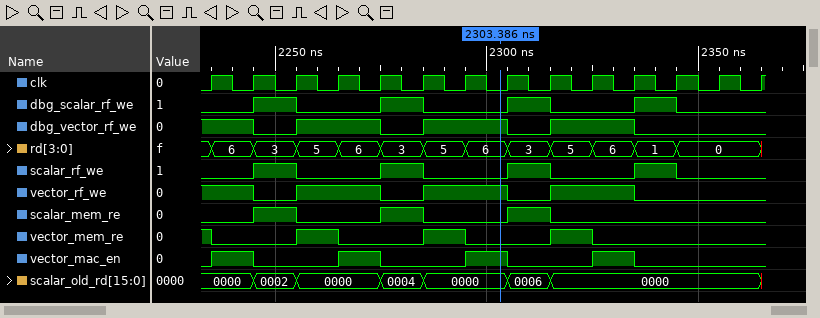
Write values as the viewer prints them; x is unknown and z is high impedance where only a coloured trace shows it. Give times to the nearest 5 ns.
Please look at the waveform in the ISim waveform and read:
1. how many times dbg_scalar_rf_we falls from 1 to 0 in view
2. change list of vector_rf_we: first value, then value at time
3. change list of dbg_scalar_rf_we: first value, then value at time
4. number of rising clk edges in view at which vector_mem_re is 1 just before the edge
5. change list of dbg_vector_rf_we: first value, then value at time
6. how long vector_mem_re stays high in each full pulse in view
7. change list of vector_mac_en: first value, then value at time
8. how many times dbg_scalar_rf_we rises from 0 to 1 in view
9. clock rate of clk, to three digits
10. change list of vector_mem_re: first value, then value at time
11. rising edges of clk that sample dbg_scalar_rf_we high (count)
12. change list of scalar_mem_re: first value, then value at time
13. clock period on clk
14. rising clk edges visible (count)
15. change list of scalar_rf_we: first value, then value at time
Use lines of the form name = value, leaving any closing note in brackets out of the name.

how many times dbg_scalar_rf_we falls from 1 to 0 in view = 4
change list of vector_rf_we: first value, then value at time = 1, 0 at 2245 ns, 1 at 2255 ns, 0 at 2275 ns, 1 at 2285 ns, 0 at 2305 ns, 1 at 2315 ns, 0 at 2335 ns
change list of dbg_scalar_rf_we: first value, then value at time = 0, 1 at 2245 ns, 0 at 2255 ns, 1 at 2275 ns, 0 at 2285 ns, 1 at 2305 ns, 0 at 2315 ns, 1 at 2335 ns, 0 at 2345 ns
number of rising clk edges in view at which vector_mem_re is 1 just before the edge = 4
change list of dbg_vector_rf_we: first value, then value at time = 1, 0 at 2245 ns, 1 at 2255 ns, 0 at 2275 ns, 1 at 2285 ns, 0 at 2305 ns, 1 at 2315 ns, 0 at 2335 ns
how long vector_mem_re stays high in each full pulse in view = 10 ns, 10 ns, 10 ns
change list of vector_mac_en: first value, then value at time = 0, 1 at 2235 ns, 0 at 2245 ns, 1 at 2265 ns, 0 at 2275 ns, 1 at 2295 ns, 0 at 2305 ns, 1 at 2325 ns, 0 at 2335 ns
how many times dbg_scalar_rf_we rises from 0 to 1 in view = 4
clock rate of clk, to three digits = 100 MHz
change list of vector_mem_re: first value, then value at time = 1, 0 at 2235 ns, 1 at 2255 ns, 0 at 2265 ns, 1 at 2285 ns, 0 at 2295 ns, 1 at 2315 ns, 0 at 2325 ns
rising edges of clk that sample dbg_scalar_rf_we high = 4
change list of scalar_mem_re: first value, then value at time = 0, 1 at 2245 ns, 0 at 2255 ns, 1 at 2275 ns, 0 at 2285 ns, 1 at 2305 ns, 0 at 2315 ns
clock period on clk = 10 ns
rising clk edges visible = 14
change list of scalar_rf_we: first value, then value at time = 0, 1 at 2245 ns, 0 at 2255 ns, 1 at 2275 ns, 0 at 2285 ns, 1 at 2305 ns, 0 at 2315 ns, 1 at 2335 ns, 0 at 2345 ns
